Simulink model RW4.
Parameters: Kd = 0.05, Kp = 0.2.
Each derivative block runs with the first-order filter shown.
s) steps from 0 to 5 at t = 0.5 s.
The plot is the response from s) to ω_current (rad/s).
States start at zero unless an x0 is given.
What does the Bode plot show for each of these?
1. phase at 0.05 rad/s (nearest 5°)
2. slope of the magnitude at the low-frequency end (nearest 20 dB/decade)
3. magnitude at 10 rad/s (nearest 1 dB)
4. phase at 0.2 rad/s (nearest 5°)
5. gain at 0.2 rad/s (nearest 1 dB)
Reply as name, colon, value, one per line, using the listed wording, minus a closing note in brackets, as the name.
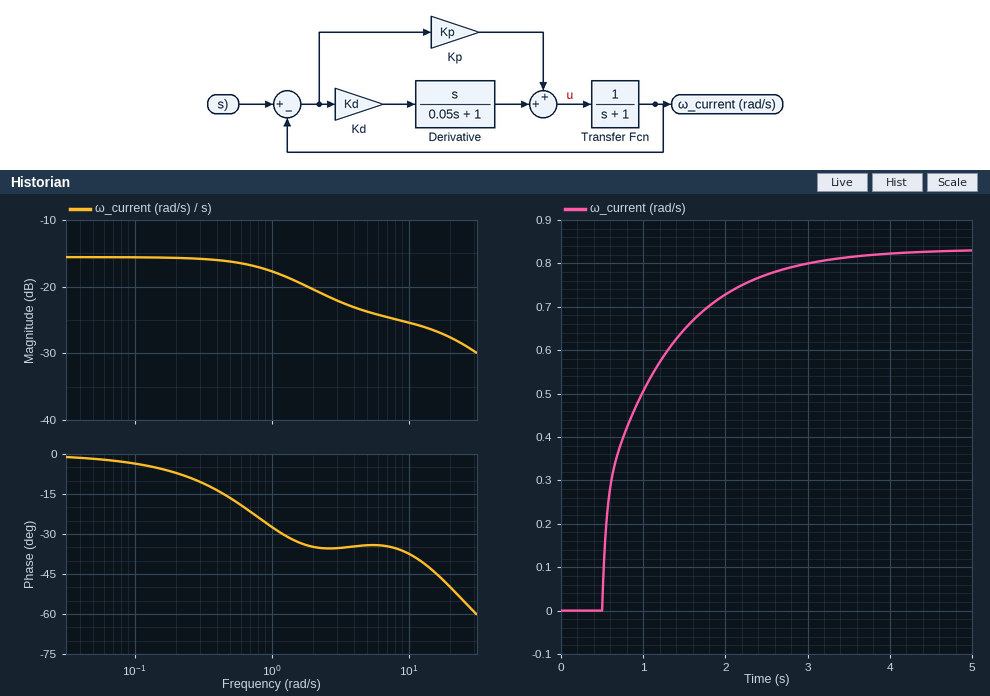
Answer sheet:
phase at 0.05 rad/s: 0°
slope of the magnitude at the low-frequency end: 0 dB/decade
magnitude at 10 rad/s: -25 dB
phase at 0.2 rad/s: -5°
gain at 0.2 rad/s: -16 dB
